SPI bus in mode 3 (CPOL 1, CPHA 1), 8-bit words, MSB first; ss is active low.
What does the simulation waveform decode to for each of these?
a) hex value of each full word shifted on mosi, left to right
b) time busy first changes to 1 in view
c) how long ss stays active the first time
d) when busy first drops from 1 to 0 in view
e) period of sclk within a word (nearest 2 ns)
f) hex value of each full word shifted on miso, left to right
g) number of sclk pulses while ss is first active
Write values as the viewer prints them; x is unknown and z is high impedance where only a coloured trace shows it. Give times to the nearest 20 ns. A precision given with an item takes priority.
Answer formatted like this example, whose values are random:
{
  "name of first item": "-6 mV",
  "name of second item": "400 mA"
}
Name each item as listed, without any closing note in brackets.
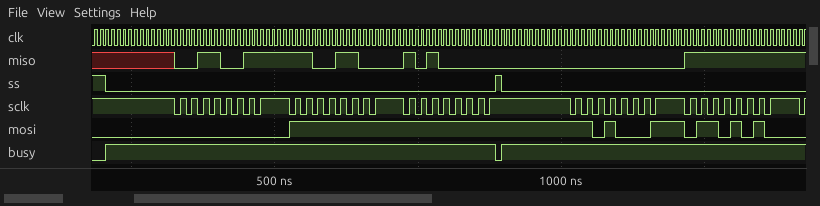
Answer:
{
  "hex value of each full word shifted on mosi, left to right": "00, FF, FF, D1, 6A",
  "time busy first changes to 1 in view": "200 ns",
  "how long ss stays active the first time": "680 ns",
  "when busy first drops from 1 to 0 in view": "880 ns",
  "period of sclk within a word": "20 ns",
  "hex value of each full word shifted on miso, left to right": "33, CC, A0, 00, FF",
  "number of sclk pulses while ss is first active": "24"
}
